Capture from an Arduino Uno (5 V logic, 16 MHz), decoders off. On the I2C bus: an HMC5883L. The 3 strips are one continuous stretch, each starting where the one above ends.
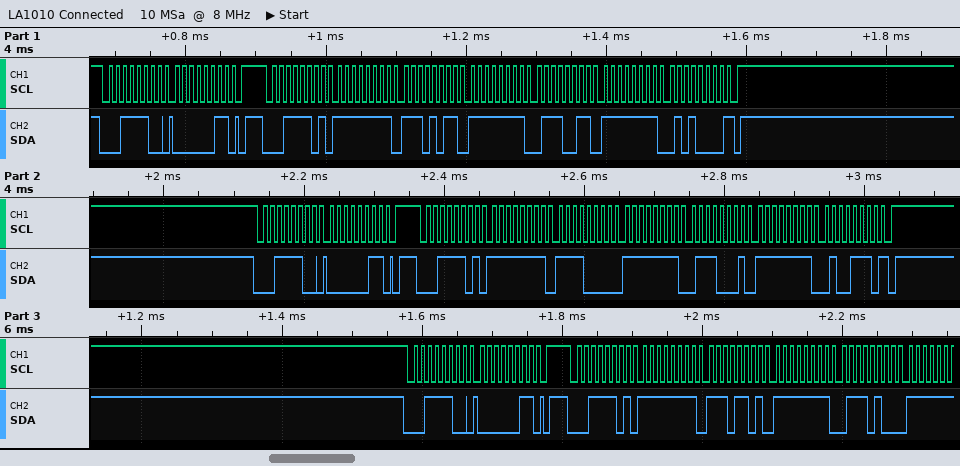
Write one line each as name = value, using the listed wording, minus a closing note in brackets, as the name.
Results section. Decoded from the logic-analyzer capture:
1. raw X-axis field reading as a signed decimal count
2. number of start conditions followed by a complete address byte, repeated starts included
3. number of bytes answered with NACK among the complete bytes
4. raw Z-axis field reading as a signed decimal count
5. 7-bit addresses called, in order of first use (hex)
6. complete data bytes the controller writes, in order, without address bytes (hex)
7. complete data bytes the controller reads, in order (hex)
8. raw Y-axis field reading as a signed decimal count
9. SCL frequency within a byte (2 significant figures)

raw X-axis field reading as a signed decimal count = -21
number of start conditions followed by a complete address byte, repeated starts included = 6
number of bytes answered with NACK among the complete bytes = 2
raw Z-axis field reading as a signed decimal count = -141
7-bit addresses called, in order of first use = 0x1E
complete data bytes the controller writes, in order, without address bytes = 03 03 03
complete data bytes the controller reads, in order = FF EB FF 73 FF 50 FF F0 FF 71 FF 4E FF ED FF 74
raw Y-axis field reading as a signed decimal count = -176
SCL frequency within a byte = 100 kHz
